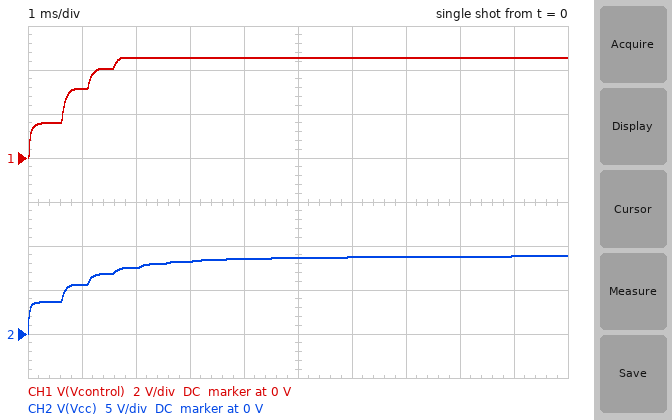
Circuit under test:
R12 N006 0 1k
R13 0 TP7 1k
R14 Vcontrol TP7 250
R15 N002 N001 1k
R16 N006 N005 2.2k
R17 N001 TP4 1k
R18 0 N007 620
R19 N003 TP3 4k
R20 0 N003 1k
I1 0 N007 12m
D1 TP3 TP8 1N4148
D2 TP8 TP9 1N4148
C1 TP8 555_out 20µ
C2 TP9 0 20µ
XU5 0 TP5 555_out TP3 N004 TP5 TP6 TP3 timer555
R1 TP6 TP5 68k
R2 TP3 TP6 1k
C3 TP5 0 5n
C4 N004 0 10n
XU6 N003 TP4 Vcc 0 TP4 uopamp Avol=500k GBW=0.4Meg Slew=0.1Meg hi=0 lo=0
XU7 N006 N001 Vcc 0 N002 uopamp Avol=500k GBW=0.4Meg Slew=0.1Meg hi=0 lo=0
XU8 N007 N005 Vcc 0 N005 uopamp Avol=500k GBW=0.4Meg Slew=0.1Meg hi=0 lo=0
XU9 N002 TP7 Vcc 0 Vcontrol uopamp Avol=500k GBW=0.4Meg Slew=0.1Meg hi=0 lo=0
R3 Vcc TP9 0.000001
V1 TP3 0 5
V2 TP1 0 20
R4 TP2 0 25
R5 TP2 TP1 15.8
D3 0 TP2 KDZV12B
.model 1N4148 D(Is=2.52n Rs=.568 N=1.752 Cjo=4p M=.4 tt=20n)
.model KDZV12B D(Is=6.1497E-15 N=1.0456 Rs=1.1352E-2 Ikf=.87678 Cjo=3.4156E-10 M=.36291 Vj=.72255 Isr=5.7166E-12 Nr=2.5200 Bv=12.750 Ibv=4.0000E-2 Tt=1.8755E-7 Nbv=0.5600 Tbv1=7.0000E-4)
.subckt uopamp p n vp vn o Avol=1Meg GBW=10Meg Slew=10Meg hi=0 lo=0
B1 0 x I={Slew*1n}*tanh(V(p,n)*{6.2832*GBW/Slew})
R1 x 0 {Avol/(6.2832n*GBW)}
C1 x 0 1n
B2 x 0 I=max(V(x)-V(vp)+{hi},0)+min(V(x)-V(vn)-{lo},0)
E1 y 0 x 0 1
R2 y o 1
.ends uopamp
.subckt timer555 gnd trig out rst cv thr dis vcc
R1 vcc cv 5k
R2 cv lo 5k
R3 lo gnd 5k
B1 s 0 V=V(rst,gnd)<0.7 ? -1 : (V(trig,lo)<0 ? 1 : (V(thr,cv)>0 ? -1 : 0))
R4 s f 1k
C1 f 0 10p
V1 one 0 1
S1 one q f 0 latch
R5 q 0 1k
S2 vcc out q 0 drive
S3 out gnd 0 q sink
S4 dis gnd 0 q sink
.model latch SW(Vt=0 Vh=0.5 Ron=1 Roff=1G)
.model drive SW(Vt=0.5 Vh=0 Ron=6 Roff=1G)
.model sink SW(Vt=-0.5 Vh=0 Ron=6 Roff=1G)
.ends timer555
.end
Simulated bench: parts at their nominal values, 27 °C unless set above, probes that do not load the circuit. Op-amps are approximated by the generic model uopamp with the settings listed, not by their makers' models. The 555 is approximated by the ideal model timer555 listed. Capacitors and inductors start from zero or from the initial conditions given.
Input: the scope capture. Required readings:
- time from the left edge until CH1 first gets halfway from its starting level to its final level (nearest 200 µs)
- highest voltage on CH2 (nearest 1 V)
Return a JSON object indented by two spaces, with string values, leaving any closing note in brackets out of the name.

{
  "time from the left edge until CH1 first gets halfway from its starting level to its final level": "600 µs",
  "highest voltage on CH2": "9 V"
}
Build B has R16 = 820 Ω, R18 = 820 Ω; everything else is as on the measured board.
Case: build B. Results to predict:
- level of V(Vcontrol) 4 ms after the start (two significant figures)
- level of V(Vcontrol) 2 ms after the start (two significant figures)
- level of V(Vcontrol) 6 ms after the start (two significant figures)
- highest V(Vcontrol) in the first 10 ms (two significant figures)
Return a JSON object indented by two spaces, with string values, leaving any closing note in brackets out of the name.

{
  "level of V(Vcontrol) 4 ms after the start": "8.5 V",
  "level of V(Vcontrol) 2 ms after the start": "7.5 V",
  "level of V(Vcontrol) 6 ms after the start": "8.7 V",
  "highest V(Vcontrol) in the first 10 ms": "8.8 V"
}
